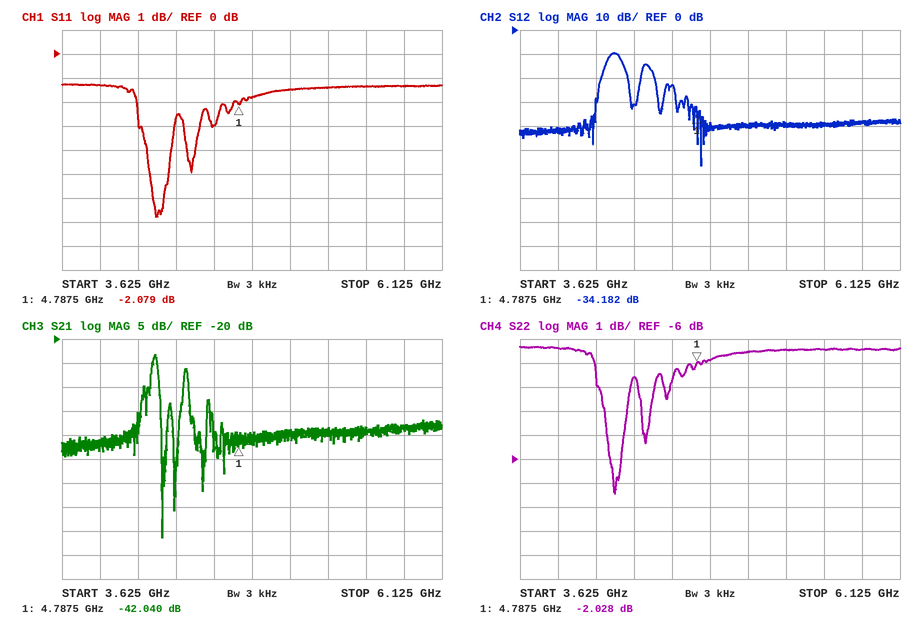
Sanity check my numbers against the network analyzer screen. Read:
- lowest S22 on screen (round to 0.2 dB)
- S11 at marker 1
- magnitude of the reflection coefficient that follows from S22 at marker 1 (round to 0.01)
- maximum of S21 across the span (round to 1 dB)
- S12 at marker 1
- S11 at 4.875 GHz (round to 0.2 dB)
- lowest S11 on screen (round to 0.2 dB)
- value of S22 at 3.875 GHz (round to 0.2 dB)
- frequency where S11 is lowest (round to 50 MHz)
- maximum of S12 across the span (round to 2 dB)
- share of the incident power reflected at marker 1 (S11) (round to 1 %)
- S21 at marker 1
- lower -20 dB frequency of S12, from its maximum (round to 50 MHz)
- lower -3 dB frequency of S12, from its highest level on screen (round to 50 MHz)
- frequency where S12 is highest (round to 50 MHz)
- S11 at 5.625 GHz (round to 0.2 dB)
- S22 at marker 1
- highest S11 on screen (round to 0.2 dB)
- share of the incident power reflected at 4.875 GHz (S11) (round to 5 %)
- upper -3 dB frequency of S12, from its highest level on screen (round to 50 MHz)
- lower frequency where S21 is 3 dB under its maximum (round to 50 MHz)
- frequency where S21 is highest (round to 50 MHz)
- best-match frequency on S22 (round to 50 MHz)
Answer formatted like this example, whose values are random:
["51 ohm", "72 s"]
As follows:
["-7.4 dB", "-2.079 dB", "0.79", "-23 dB", "-34.182 dB", "-1.8 dB", "-6.8 dB", "-1.4 dB", "4.25 GHz", "-10 dB", "62 %", "-42.040 dB", "4.15 GHz", "4.20 GHz", "4.25 GHz", "-1.4 dB", "-2.028 dB", "-1.2 dB", "65 %", "4.30 GHz", "4.20 GHz", "4.25 GHz", "4.25 GHz"]
